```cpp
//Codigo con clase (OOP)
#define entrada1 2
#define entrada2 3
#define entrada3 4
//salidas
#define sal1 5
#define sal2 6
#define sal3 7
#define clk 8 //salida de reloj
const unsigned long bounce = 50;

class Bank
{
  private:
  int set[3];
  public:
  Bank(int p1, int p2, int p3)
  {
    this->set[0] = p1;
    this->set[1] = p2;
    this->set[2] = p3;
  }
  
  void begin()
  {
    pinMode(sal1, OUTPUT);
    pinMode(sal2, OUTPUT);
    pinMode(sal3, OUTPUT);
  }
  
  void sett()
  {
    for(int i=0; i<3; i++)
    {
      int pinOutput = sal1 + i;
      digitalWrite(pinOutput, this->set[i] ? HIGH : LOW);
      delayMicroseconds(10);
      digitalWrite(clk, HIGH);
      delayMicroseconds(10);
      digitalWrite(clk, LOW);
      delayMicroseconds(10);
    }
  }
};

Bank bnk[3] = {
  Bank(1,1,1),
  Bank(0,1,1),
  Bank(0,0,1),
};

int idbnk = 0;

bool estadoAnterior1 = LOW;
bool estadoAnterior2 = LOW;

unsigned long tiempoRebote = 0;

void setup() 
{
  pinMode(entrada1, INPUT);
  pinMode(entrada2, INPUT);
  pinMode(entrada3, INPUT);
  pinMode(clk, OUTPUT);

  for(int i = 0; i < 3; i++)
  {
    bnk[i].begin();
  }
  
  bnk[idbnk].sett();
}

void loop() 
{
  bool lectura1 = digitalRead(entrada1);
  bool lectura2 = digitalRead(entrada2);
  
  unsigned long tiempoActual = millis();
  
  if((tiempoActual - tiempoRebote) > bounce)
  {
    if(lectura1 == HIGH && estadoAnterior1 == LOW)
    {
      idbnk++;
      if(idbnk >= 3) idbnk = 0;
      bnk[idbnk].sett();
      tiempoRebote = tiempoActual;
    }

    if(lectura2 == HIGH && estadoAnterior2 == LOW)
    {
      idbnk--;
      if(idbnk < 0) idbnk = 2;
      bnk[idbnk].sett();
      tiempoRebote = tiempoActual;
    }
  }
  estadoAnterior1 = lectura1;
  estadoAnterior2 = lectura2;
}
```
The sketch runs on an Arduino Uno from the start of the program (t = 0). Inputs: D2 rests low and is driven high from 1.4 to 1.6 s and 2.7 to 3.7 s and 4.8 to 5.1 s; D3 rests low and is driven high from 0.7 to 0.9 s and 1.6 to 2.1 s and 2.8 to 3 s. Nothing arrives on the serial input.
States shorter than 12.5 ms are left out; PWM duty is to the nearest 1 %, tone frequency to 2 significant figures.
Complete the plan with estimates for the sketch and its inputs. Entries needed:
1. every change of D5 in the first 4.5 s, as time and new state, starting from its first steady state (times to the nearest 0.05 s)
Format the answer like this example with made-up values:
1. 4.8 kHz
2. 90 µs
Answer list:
1. 0 s high; 0.7 s low; 1.4 s high; 1.6 s low; 2.7 s high; 2.8 s low
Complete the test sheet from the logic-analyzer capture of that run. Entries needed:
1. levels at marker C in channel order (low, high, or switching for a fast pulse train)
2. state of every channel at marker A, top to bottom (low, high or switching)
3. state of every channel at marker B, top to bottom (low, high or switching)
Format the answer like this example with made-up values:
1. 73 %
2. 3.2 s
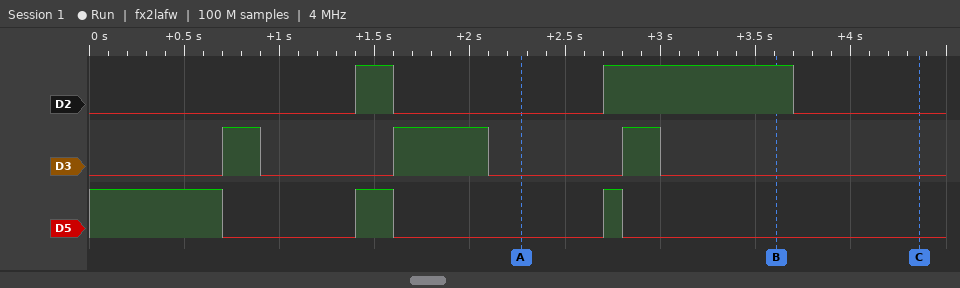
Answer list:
1. D2 low, D3 low, D5 low
2. D2 low, D3 low, D5 low
3. D2 high, D3 low, D5 low
